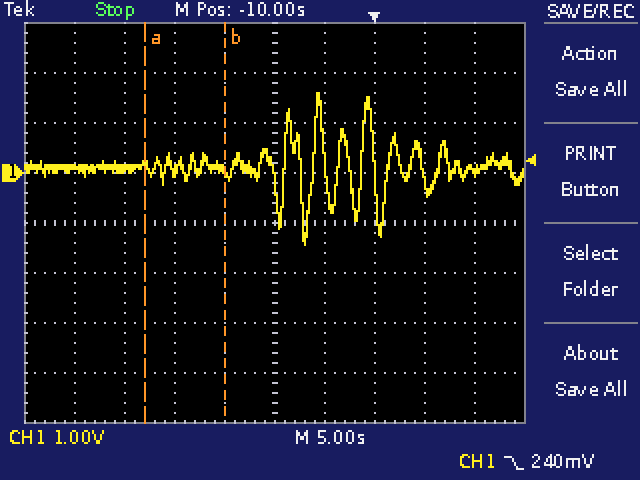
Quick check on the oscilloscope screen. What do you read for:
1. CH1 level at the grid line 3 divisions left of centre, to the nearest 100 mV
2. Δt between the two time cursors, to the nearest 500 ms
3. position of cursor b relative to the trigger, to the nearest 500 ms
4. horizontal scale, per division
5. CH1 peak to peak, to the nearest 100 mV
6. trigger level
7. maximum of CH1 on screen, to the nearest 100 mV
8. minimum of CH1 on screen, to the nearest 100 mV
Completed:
100 mV
8.0 s
-15.0 s
5 s
3.0 V
240 mV
1.6 V
-1.4 V
